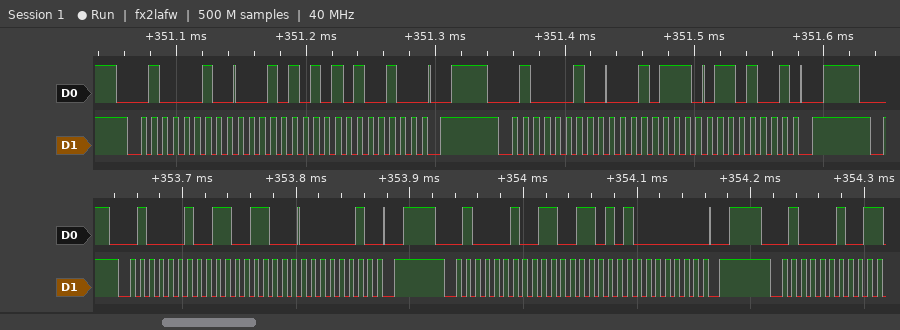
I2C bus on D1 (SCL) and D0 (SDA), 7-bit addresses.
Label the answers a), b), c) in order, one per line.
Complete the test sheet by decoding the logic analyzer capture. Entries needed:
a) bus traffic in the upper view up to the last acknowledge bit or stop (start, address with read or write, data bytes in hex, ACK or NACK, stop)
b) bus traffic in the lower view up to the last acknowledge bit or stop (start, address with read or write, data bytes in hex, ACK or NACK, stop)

a) start, address 21 write ACK, 15 ACK, A4 ACK, stop, start, address 21 write ACK, 17 ACK, 69 ACK, stop
b) start, address 21 write ACK, CC ACK, 02 ACK, stop, start, address 21 write ACK, CD ACK, 80 ACK, stop, start, address 21 write ACK
